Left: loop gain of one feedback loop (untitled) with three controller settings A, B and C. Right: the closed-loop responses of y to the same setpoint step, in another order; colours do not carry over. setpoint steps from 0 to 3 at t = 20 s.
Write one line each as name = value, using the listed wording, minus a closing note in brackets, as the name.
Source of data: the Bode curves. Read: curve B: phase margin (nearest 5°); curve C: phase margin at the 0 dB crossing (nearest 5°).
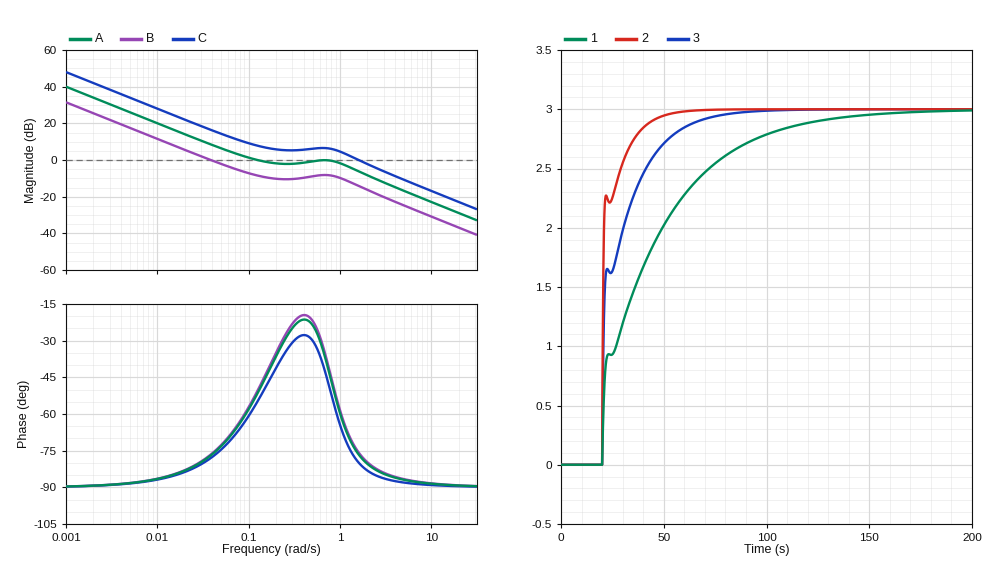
curve B: phase margin = 105°
curve C: phase margin at the 0 dB crossing = 100°
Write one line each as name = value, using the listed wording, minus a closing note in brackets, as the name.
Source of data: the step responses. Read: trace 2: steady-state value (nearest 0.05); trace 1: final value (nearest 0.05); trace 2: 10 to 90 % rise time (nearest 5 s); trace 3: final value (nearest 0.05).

trace 2: steady-state value = 3.00
trace 1: final value = 3.00
trace 2: 10 to 90 % rise time = 15 s
trace 3: final value = 3.00
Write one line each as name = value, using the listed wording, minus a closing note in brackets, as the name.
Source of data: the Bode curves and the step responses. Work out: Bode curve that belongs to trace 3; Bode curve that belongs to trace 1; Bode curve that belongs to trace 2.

Bode curve that belongs to trace 3 = A
Bode curve that belongs to trace 1 = B
Bode curve that belongs to trace 2 = C
